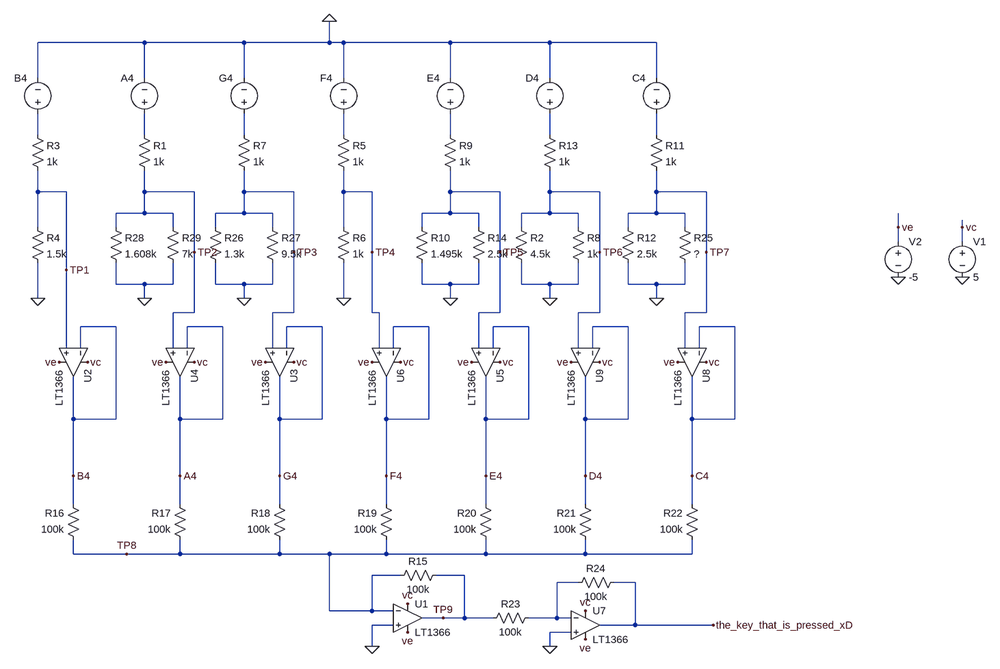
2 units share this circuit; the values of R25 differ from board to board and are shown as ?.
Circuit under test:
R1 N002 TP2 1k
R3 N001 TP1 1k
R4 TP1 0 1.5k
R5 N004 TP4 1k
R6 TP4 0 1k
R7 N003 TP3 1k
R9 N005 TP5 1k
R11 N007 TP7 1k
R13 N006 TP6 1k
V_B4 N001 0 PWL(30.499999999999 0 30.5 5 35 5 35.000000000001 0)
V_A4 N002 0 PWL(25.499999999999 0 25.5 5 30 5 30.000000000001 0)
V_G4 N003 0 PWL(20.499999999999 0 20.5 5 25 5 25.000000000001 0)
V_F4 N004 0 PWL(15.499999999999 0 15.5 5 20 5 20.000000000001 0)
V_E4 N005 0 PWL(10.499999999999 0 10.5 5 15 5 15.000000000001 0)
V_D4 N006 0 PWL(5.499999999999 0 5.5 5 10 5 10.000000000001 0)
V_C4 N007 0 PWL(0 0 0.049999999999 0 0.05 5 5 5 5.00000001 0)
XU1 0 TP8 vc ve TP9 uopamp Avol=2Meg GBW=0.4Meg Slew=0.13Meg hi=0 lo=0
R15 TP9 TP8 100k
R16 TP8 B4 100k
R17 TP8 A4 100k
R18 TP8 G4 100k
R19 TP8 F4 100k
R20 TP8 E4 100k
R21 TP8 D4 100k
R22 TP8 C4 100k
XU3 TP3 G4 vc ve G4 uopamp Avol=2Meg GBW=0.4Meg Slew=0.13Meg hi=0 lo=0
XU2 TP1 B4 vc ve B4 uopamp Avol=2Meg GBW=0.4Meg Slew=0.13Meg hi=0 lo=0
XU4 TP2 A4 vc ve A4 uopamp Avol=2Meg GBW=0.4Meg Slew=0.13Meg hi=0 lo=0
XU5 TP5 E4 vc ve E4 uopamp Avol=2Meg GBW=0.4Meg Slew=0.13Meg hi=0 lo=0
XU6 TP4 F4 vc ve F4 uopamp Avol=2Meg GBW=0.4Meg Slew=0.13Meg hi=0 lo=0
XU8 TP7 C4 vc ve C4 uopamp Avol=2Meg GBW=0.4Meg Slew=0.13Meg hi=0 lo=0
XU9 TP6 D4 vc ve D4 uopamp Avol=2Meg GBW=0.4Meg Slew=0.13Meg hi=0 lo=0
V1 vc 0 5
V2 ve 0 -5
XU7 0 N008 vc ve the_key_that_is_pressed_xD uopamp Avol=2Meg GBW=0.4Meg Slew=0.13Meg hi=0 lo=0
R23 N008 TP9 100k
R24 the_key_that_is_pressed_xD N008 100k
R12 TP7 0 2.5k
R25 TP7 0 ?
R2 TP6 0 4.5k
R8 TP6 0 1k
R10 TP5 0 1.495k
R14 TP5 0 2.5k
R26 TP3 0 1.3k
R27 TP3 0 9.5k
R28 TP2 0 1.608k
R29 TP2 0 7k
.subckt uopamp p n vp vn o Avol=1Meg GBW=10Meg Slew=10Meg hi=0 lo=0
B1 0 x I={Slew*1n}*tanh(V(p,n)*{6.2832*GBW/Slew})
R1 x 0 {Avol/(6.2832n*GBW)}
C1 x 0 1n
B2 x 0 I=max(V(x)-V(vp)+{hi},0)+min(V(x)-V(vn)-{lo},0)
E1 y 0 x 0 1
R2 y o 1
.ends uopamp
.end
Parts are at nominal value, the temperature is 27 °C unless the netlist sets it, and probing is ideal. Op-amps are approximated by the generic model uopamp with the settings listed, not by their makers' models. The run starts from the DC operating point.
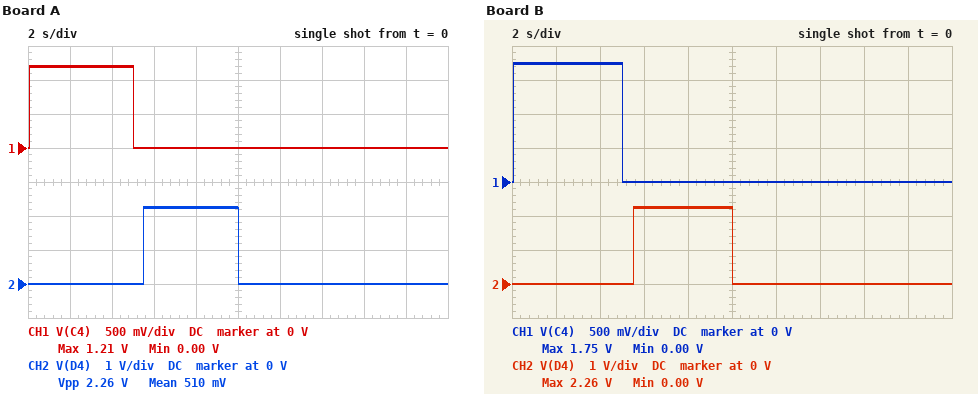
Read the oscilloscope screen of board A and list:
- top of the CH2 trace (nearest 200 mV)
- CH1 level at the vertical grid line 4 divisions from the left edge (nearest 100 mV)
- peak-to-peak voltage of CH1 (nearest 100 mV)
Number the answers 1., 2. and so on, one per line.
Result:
1. 2.2 V
2. 0 V
3. 1.2 V
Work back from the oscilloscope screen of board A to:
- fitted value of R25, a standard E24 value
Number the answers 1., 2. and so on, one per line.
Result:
1. 360 Ω
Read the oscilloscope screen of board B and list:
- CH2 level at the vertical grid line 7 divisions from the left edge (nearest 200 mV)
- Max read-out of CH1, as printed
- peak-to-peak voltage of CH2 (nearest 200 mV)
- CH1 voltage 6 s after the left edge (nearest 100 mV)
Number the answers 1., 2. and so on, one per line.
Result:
1. 0 V
2. 1.75 V
3. 2.2 V
4. 0 V
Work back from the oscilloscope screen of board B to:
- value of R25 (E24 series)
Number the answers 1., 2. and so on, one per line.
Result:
1. 680 Ω
